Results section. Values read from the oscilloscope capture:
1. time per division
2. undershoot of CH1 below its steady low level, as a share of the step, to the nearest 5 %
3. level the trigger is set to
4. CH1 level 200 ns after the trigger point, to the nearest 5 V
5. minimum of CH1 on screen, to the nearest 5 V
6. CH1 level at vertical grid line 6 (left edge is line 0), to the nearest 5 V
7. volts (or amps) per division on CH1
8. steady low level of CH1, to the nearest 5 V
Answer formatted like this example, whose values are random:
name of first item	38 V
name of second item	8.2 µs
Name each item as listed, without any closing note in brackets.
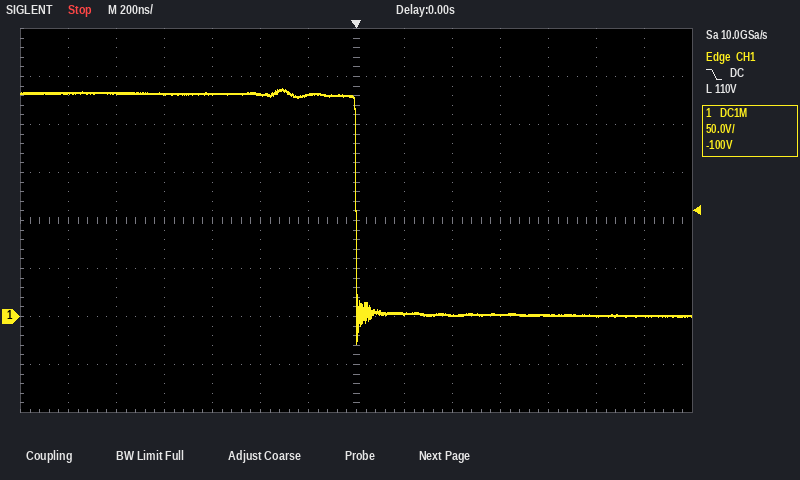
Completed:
time per division	200 ns
undershoot of CH1 below its steady low level, as a share of the step, to the nearest 5 %	15 %
level the trigger is set to	110 V
CH1 level 200 ns after the trigger point, to the nearest 5 V	5 V
minimum of CH1 on screen, to the nearest 5 V	-30 V
CH1 level at vertical grid line 6 (left edge is line 0), to the nearest 5 V	230 V
volts (or amps) per division on CH1	50 V
steady low level of CH1, to the nearest 5 V	0 V
